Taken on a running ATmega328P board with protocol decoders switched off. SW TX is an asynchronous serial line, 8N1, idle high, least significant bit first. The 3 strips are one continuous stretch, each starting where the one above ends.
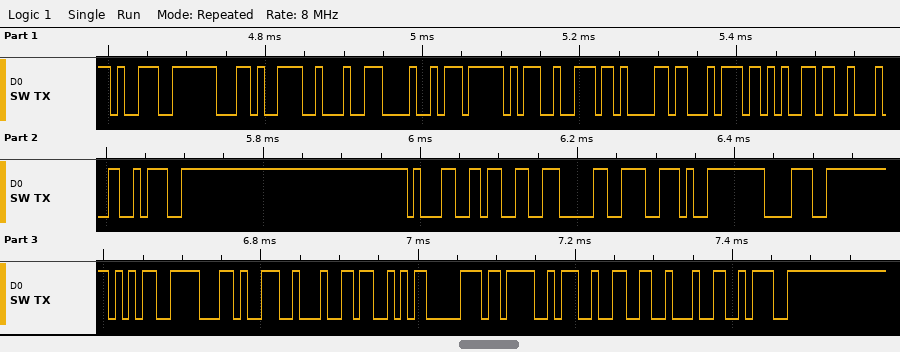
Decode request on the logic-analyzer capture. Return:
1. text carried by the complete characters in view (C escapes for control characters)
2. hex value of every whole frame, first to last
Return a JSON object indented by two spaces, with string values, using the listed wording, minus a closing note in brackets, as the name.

{
  "text carried by the complete characters in view": "\"9,\\\"H_rate\\\":130.85,\\\"SpO2\\\":\"",
  "hex value of every whole frame, first to last": "39 2C 22 48 5F 72 61 74 65 22 3A 31 33 30 2E 38 35 2C 22 53 70 4F 32 22 3A"
}
